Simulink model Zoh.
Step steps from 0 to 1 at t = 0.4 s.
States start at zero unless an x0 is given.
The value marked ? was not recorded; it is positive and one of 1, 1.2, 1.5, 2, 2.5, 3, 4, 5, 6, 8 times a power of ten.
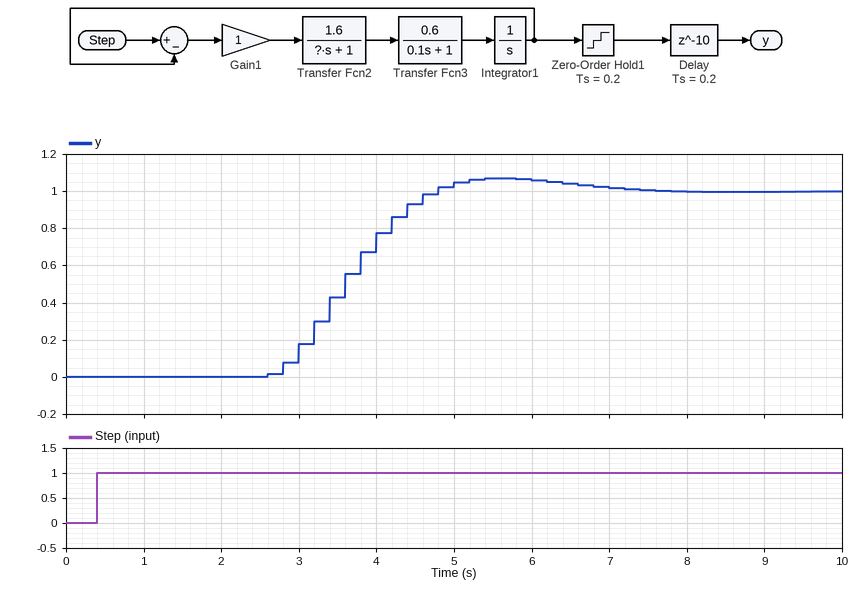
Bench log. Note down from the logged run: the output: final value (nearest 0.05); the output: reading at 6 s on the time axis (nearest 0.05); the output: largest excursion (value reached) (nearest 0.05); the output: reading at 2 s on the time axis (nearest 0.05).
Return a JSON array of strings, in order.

["1.00", "1.05", "1.05", "0.00"]
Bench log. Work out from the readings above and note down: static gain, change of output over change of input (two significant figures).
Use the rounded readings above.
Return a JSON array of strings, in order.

["1.0"]
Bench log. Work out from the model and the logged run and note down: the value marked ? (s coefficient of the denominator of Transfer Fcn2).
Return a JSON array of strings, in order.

["0.5"]
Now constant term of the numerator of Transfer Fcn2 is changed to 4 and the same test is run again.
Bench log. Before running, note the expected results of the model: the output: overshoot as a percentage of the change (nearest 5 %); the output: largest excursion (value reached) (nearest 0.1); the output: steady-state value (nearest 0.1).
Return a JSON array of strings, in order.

["30 %", "1.3", "1.0"]
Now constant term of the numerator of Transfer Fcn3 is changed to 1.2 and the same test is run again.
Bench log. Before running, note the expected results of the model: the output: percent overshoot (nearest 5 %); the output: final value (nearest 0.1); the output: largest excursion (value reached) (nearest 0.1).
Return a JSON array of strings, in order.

["25 %", "1.0", "1.2"]
